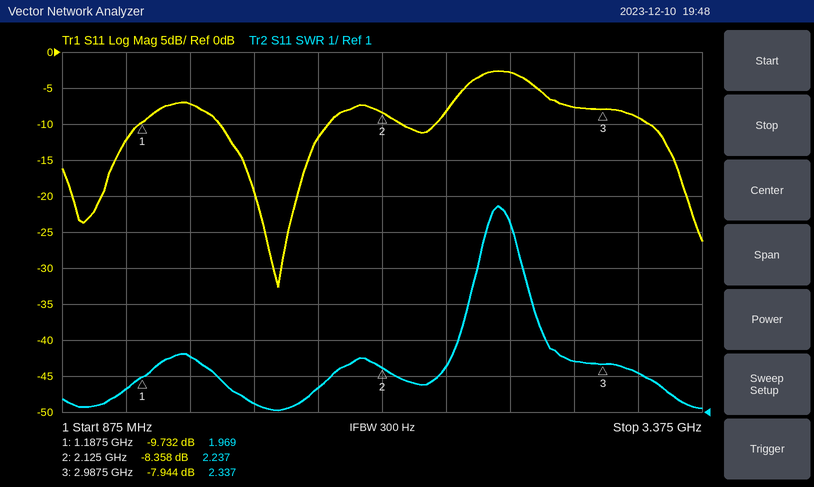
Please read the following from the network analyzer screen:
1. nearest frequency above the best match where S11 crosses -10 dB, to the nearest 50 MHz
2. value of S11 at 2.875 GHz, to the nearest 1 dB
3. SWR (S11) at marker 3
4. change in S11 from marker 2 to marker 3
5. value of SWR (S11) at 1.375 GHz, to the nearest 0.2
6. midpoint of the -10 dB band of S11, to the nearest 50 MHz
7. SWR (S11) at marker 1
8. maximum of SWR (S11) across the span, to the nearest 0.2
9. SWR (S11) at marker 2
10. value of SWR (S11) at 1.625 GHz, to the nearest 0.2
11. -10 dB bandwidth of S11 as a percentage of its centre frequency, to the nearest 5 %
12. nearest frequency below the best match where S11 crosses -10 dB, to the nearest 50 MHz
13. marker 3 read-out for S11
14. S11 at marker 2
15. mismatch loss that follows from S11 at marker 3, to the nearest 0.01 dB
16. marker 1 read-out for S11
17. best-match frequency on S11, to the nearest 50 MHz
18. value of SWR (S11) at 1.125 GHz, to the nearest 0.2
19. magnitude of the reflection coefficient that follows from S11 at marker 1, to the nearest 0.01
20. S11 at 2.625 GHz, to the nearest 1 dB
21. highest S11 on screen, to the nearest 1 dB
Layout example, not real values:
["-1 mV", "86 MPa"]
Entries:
["1.90 GHz", "-8 dB", "2.337", "0.414 dB", "2.6", "1.70 GHz", "1.969", "6.8", "2.237", "1.2", "25 %", "1.50 GHz", "-7.944 dB", "-8.358 dB", "0.76 dB", "-9.732 dB", "1.70 GHz", "1.6", "0.33", "-3 dB", "-3 dB"]
